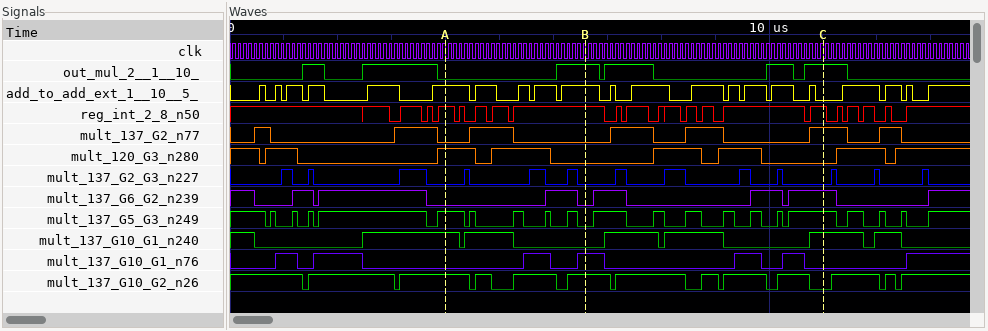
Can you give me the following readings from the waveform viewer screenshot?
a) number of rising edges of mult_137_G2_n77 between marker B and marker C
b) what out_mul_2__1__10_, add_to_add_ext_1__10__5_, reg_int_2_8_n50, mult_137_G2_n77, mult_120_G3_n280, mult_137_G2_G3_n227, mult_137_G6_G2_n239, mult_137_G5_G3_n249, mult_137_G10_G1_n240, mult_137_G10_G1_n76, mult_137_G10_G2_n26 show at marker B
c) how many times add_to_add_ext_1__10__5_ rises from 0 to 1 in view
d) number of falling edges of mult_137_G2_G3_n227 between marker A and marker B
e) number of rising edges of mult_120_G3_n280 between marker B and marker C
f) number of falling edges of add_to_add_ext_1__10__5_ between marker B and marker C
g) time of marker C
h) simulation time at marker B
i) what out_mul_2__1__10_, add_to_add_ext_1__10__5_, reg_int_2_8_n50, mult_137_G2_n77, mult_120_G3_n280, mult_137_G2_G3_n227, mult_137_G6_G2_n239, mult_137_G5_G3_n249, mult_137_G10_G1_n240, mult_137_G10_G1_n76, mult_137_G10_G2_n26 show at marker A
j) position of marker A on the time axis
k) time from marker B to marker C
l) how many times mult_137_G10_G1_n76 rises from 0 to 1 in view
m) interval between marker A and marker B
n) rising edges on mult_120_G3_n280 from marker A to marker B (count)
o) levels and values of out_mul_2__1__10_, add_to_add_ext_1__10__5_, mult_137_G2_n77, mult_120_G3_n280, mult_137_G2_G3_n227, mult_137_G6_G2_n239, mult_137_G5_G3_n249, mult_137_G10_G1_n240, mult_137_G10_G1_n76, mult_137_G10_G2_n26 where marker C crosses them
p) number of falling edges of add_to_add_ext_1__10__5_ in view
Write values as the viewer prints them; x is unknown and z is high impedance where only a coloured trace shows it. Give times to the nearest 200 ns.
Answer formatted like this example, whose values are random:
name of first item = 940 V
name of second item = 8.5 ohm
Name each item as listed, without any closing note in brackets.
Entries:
number of rising edges of mult_137_G2_n77 between marker B and marker C = 3
what out_mul_2__1__10_, add_to_add_ext_1__10__5_, reg_int_2_8_n50, mult_137_G2_n77, mult_120_G3_n280, mult_137_G2_G3_n227, mult_137_G6_G2_n239, mult_137_G5_G3_n249, mult_137_G10_G1_n240, mult_137_G10_G1_n76, mult_137_G10_G2_n26 show at marker B = out_mul_2__1__10_=1, add_to_add_ext_1__10__5_=1, reg_int_2_8_n50=1, mult_137_G2_n77=0, mult_120_G3_n280=0, mult_137_G2_G3_n227=0, mult_137_G6_G2_n239=0, mult_137_G5_G3_n249=0, mult_137_G10_G1_n240=0, mult_137_G10_G1_n76=1, mult_137_G10_G2_n26=1
how many times add_to_add_ext_1__10__5_ rises from 0 to 1 in view = 21
number of falling edges of mult_137_G2_G3_n227 between marker A and marker B = 3
number of rising edges of mult_120_G3_n280 between marker B and marker C = 2
number of falling edges of add_to_add_ext_1__10__5_ between marker B and marker C = 8
time of marker C = 11000 ns
simulation time at marker B = 6600 ns
what out_mul_2__1__10_, add_to_add_ext_1__10__5_, reg_int_2_8_n50, mult_137_G2_n77, mult_120_G3_n280, mult_137_G2_G3_n227, mult_137_G6_G2_n239, mult_137_G5_G3_n249, mult_137_G10_G1_n240, mult_137_G10_G1_n76, mult_137_G10_G2_n26 show at marker A = out_mul_2__1__10_=0, add_to_add_ext_1__10__5_=1, reg_int_2_8_n50=1, mult_137_G2_n77=0, mult_120_G3_n280=1, mult_137_G2_G3_n227=0, mult_137_G6_G2_n239=0, mult_137_G5_G3_n249=1, mult_137_G10_G1_n240=1, mult_137_G10_G1_n76=0, mult_137_G10_G2_n26=1
position of marker A on the time axis = 4000 ns
time from marker B to marker C = 4400 ns
how many times mult_137_G10_G1_n76 rises from 0 to 1 in view = 7
interval between marker A and marker B = 2600 ns
rising edges on mult_120_G3_n280 from marker A to marker B = 1
levels and values of out_mul_2__1__10_, add_to_add_ext_1__10__5_, mult_137_G2_n77, mult_120_G3_n280, mult_137_G2_G3_n227, mult_137_G6_G2_n239, mult_137_G5_G3_n249, mult_137_G10_G1_n240, mult_137_G10_G1_n76, mult_137_G10_G2_n26 where marker C crosses them = out_mul_2__1__10_=1, add_to_add_ext_1__10__5_=0, mult_137_G2_n77=1, mult_120_G3_n280=0, mult_137_G2_G3_n227=0, mult_137_G6_G2_n239=1, mult_137_G5_G3_n249=1, mult_137_G10_G1_n240=1, mult_137_G10_G1_n76=0, mult_137_G10_G2_n26=0
number of falling edges of add_to_add_ext_1__10__5_ in view = 20
